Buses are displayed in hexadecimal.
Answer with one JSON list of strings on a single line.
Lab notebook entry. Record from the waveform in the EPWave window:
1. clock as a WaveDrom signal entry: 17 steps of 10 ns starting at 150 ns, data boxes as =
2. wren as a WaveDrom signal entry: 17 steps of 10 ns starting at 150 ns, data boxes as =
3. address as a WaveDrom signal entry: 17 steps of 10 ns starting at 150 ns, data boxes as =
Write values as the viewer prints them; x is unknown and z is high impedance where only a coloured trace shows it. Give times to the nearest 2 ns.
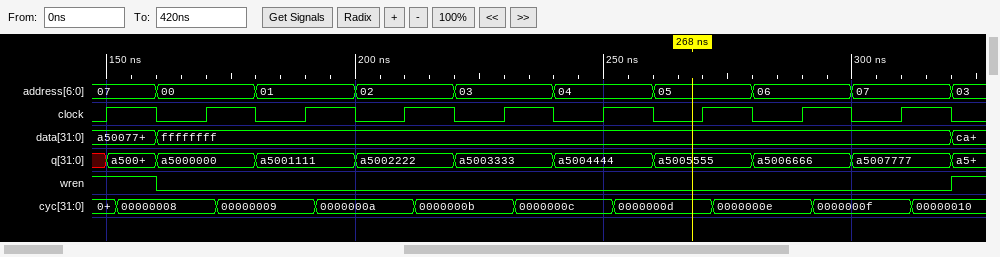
["{name: 'clock', wave: '10101010101010101'}", "{name: 'wren', wave: '10...............'}", "{name: 'address', wave: '==.=.=.=.=.=.=.=.', data: '07 00 01 02 03 04 05 06 07'}"]
